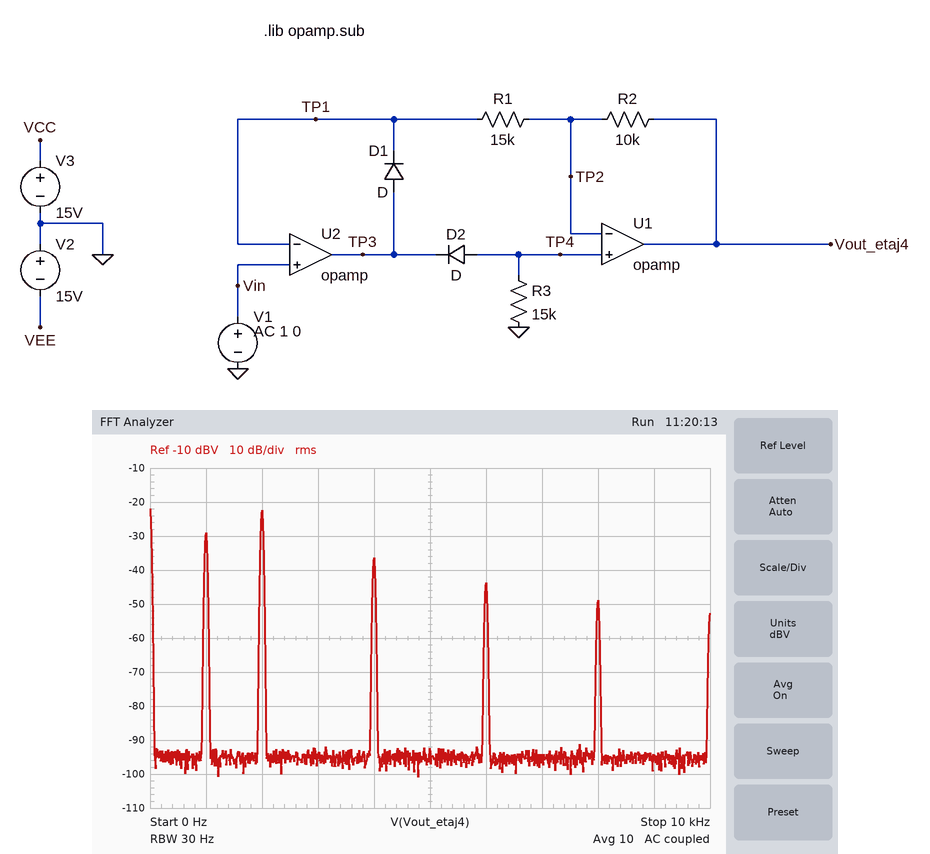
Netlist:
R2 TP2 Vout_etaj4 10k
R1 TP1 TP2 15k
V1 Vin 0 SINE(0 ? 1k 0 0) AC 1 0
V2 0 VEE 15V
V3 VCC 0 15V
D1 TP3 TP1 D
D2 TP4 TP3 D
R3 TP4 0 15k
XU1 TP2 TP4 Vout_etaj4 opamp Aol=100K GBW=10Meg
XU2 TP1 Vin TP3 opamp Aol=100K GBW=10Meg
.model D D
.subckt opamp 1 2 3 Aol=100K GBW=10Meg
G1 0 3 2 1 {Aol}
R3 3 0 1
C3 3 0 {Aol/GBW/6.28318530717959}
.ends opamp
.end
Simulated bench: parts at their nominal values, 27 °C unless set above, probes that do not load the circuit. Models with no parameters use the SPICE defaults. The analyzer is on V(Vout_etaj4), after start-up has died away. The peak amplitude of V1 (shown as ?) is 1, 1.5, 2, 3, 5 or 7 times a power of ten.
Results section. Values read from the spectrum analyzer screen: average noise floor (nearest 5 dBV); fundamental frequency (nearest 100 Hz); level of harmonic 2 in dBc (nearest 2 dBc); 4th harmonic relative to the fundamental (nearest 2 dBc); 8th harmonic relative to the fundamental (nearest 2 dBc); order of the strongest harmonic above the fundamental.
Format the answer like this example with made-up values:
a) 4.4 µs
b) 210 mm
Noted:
a) -95 dBV
b) 1.0 kHz
c) 6 dBc
d) -8 dBc
e) -20 dBc
f) 2
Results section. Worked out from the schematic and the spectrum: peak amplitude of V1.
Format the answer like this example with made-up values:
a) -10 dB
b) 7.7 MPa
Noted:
a) 300 mV
